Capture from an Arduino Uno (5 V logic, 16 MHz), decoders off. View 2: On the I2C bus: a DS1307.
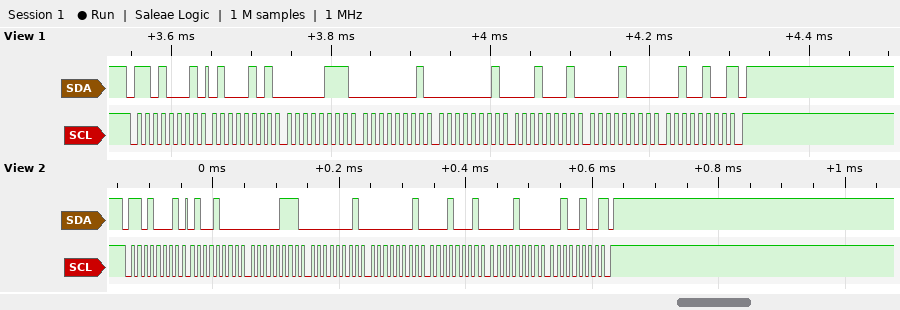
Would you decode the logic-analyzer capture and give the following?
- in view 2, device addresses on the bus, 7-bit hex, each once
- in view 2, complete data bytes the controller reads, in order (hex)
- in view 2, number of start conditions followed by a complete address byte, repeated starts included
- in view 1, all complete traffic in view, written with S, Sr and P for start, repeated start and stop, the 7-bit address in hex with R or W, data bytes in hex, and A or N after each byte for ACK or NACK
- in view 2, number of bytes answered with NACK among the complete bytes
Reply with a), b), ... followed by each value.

a) 0x68
b) 48 07 01 01 11 08 24
c) 1
d) S 68R A 45 A 07 A 01 A 01 A 11 A 08 A 24 N P
e) 1
